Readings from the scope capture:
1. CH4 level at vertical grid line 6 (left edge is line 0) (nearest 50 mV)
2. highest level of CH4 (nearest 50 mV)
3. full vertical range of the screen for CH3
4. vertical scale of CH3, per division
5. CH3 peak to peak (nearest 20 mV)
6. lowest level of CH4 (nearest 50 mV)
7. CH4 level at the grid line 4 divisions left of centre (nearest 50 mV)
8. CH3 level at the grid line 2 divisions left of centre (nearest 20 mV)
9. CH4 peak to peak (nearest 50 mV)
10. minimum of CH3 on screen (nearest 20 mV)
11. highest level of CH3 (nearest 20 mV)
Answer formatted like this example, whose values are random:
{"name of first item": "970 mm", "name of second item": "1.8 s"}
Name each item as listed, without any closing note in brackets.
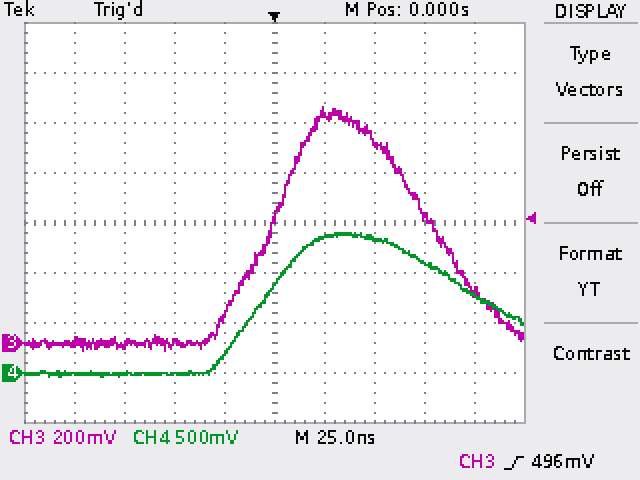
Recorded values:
{"CH4 level at vertical grid line 6 (left edge is line 0)": "1.35 V", "highest level of CH4": "1.40 V", "full vertical range of the screen for CH3": "1.6 V", "vertical scale of CH3, per division": "200 mV", "CH3 peak to peak": "980 mV", "lowest level of CH4": "-50 mV", "CH4 level at the grid line 4 divisions left of centre": "0 mV", "CH3 level at the grid line 2 divisions left of centre": "0 mV", "CH4 peak to peak": "1.45 V", "minimum of CH3 on screen": "-40 mV", "highest level of CH3": "940 mV"}
